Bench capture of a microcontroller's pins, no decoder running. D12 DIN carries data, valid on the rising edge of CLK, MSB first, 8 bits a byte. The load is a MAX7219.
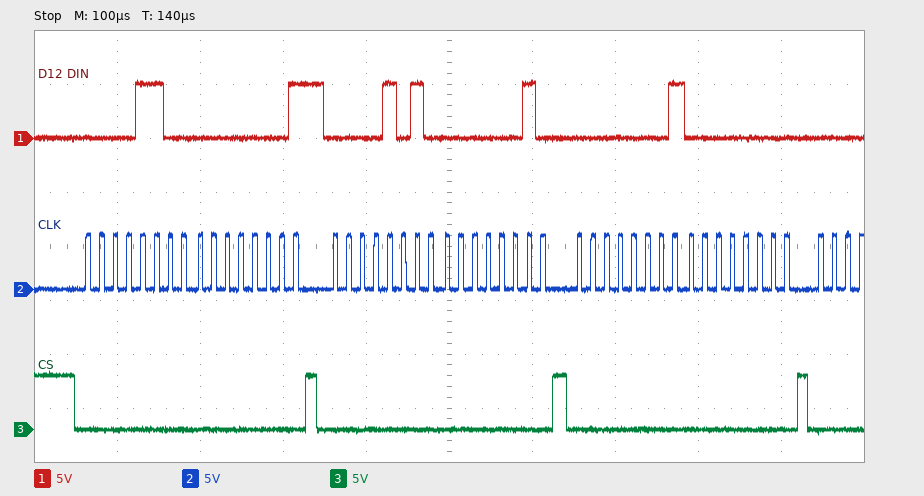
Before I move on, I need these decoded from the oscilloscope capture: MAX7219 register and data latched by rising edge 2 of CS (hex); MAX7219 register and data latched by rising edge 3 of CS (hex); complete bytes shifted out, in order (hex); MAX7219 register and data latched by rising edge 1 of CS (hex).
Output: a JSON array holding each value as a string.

["register 0xA, data 0x02", "register 0x1, data 0x00", "0C 01 0A 02 01 00", "register 0xC, data 0x01"]
